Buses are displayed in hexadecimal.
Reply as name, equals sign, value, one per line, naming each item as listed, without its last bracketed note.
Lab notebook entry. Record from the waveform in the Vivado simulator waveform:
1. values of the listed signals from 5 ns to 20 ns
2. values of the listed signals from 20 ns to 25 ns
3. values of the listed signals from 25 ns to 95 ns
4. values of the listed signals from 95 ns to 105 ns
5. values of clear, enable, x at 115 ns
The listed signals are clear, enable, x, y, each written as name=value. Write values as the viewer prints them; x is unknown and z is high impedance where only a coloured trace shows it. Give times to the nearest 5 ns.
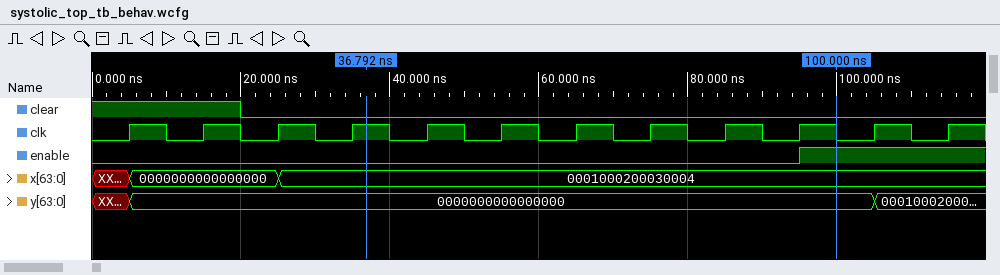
values of the listed signals from 5 ns to 20 ns = clear=1, enable=0, x=0000000000000000, y=0000000000000000
values of the listed signals from 20 ns to 25 ns = clear=0, enable=0, x=0000000000000000, y=0000000000000000
values of the listed signals from 25 ns to 95 ns = clear=0, enable=0, x=0001000200030004, y=0000000000000000
values of the listed signals from 95 ns to 105 ns = clear=0, enable=1, x=0001000200030004, y=0000000000000000
values of clear, enable, x at 115 ns = clear=0, enable=1, x=0001000200030004
